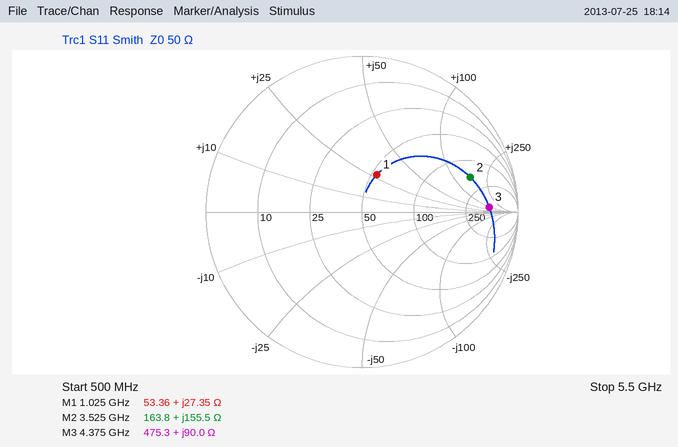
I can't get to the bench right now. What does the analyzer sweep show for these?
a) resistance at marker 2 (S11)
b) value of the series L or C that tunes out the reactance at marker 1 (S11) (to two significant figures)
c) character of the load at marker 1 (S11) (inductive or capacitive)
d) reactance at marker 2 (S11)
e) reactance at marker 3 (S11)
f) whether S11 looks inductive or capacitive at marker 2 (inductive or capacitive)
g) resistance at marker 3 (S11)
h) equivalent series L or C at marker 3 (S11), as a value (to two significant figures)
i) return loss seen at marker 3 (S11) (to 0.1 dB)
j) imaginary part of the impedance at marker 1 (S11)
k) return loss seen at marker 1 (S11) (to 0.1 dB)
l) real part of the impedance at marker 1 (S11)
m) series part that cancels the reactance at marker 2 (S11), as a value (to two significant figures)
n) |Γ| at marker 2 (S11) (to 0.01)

163.8 Ω
5.7 pF
inductive
+155.5 Ω
+90.0 Ω
inductive
475.3 Ω
3.3 nH
1.8 dB
+27.35 Ω
11.8 dB
53.36 Ω
290 fF
0.73
